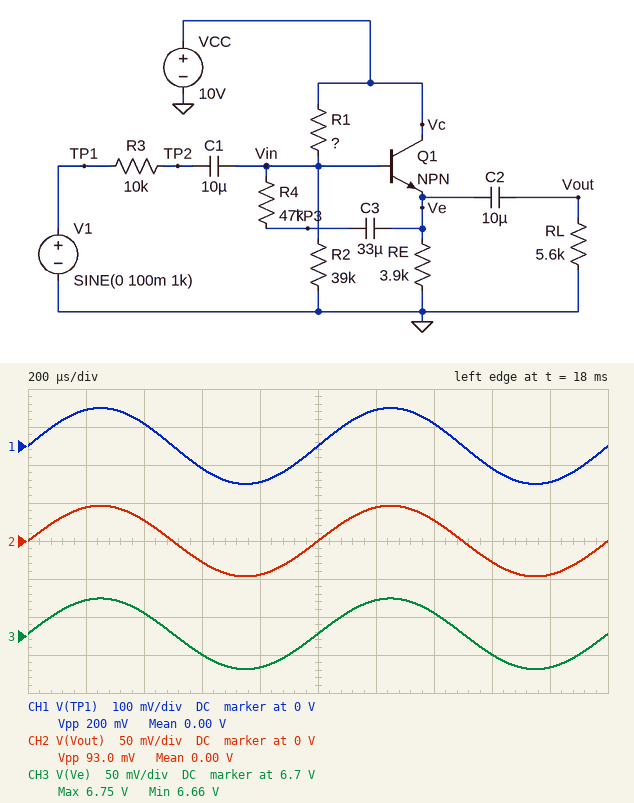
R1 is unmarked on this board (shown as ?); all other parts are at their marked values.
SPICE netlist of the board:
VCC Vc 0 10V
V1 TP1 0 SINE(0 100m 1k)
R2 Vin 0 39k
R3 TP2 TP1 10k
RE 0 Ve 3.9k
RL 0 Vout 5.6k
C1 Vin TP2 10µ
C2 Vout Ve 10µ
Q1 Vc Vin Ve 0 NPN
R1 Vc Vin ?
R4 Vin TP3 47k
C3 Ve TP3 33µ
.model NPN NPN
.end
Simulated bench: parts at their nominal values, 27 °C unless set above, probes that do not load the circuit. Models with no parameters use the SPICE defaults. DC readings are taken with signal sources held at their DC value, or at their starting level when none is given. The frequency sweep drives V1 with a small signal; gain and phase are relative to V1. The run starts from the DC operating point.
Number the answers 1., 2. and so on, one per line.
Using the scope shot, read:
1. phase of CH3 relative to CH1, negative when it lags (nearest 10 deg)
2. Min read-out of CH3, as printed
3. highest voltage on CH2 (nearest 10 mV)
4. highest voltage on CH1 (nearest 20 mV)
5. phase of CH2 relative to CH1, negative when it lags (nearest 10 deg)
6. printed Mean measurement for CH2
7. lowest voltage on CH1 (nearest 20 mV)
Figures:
1. 0 deg
2. 6.66 V
3. 50 mV
4. 100 mV
5. 0 deg
6. 0.00 V
7. -100 mV
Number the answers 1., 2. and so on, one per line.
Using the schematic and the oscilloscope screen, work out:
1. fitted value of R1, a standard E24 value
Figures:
1. 12 kΩ
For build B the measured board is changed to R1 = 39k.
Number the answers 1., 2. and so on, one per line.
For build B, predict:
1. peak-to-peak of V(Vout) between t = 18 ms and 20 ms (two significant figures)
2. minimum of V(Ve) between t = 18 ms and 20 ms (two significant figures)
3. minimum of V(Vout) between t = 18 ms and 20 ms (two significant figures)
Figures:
1. 130 mV
2. 4.0 V
3. -64 mV
